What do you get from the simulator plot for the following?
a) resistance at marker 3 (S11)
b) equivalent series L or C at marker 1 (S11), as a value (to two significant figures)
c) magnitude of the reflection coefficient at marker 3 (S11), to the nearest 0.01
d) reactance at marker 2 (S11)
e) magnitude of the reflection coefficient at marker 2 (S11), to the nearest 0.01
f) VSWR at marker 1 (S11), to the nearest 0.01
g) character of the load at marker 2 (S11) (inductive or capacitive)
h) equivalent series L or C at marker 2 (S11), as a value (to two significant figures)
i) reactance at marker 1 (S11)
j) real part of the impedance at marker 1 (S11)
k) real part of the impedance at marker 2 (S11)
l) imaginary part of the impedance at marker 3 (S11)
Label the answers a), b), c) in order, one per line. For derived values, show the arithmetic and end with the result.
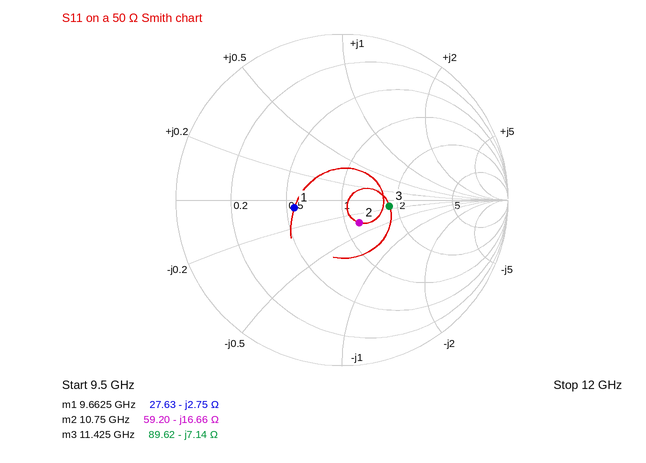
a) 89.62 Ω
b) C = 1/(2π × 9.6625 GHz × 2.75 Ω) ≈ 6.0 pF
c) 0.29
d) -16.66 Ω
e) 0.17
f) 1.82
g) capacitive
h) C = 1/(2π × 10.75 GHz × 16.66 Ω) ≈ 889 fF, so 890 fF to two significant figures
i) -2.75 Ω
j) 27.63 Ω
k) 59.20 Ω
l) -7.14 Ω
